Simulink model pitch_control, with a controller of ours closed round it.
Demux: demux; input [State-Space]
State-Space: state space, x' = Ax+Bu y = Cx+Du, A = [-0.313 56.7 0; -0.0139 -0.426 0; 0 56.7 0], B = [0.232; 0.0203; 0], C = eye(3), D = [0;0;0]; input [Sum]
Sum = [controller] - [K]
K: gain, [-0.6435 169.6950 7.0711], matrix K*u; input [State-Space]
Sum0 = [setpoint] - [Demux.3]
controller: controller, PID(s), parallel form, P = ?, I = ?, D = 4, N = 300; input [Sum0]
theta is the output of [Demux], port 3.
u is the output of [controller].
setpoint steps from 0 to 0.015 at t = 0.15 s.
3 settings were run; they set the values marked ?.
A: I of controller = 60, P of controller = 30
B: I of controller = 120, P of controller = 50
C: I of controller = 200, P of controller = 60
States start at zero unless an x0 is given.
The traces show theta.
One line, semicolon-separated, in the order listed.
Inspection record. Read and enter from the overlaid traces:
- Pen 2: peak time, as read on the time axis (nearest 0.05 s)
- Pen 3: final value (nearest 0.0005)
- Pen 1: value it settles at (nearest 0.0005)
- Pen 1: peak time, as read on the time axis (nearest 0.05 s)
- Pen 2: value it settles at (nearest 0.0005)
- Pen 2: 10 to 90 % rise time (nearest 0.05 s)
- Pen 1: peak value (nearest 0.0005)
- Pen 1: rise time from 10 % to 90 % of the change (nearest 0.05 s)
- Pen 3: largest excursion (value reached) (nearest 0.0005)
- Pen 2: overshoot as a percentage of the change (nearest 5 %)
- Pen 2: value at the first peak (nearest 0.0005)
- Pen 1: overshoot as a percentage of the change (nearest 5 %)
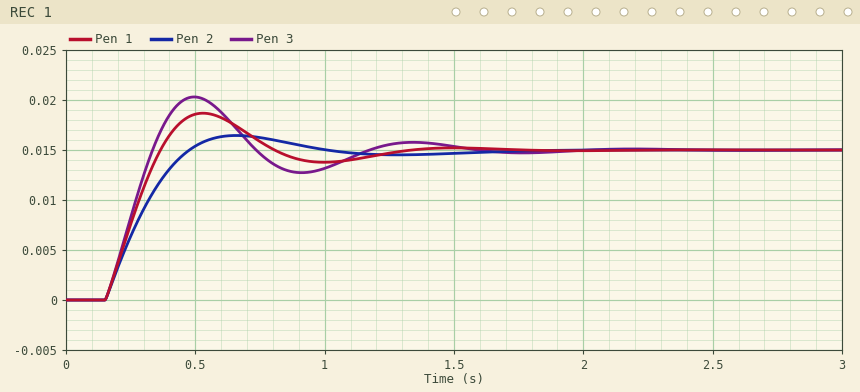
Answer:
0.65 s; 0.0150; 0.0150; 0.55 s; 0.0150; 0.25 s; 0.0185; 0.15 s; 0.0205; 10 %; 0.0165; 25 %
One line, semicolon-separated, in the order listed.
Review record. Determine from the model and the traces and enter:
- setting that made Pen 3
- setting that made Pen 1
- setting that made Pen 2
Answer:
C; B; A
